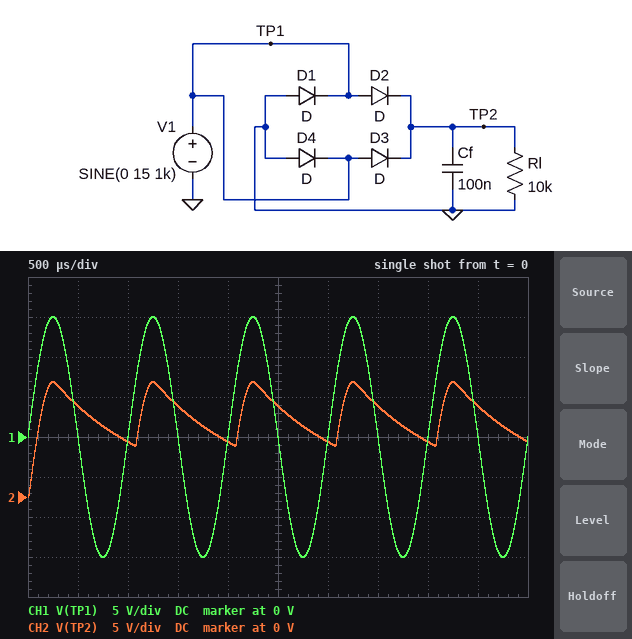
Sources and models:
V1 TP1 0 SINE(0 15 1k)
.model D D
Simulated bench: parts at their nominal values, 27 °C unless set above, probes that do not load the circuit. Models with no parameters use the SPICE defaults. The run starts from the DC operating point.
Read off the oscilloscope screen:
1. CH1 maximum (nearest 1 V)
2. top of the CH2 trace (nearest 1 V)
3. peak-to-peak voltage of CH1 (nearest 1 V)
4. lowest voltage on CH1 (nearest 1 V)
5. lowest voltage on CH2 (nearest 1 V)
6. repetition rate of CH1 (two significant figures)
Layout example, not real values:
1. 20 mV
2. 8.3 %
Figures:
1. 15 V
2. 14 V
3. 30 V
4. -15 V
5. 0 V
6. 1.0 kHz
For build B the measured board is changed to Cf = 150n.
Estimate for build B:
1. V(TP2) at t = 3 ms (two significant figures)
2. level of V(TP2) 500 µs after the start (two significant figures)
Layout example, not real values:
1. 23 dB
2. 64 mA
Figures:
1. 8.8 V
2. 12 V
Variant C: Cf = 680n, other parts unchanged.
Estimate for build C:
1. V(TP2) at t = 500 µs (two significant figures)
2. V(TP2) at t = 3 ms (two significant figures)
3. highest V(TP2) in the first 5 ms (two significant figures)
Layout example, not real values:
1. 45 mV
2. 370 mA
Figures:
1. 14 V
2. 13 V
3. 14 V
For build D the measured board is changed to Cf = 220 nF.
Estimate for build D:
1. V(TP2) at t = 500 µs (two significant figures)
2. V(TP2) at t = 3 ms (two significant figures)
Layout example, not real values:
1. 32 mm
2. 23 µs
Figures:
1. 13 V
2. 10 V
